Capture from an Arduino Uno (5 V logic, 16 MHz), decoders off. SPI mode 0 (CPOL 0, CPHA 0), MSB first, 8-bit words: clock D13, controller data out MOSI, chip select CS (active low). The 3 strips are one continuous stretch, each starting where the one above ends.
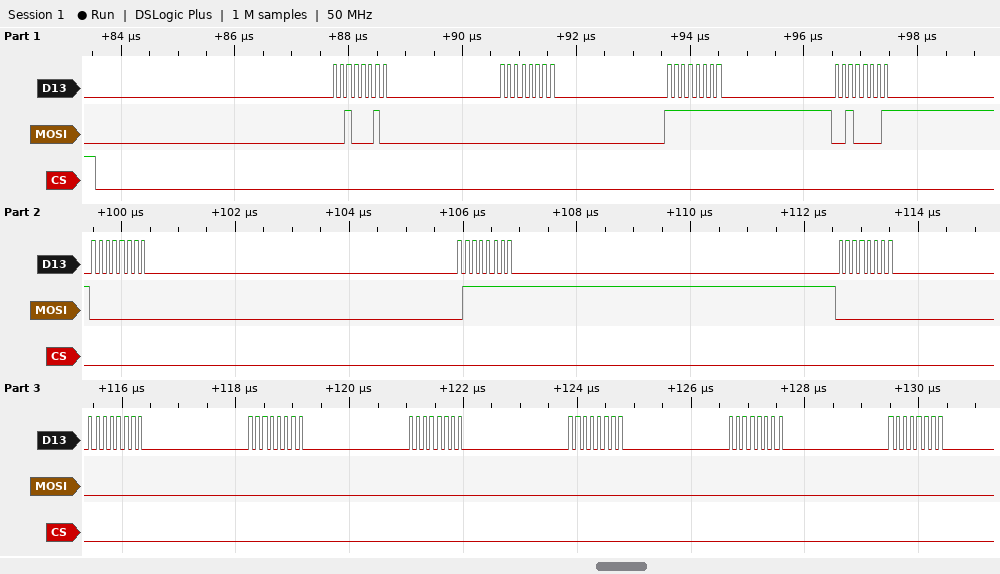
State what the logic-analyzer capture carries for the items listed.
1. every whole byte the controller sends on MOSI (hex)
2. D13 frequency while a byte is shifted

22 00 FF 21 00 7F 00 00 00 00 00 00 00
8 MHz
